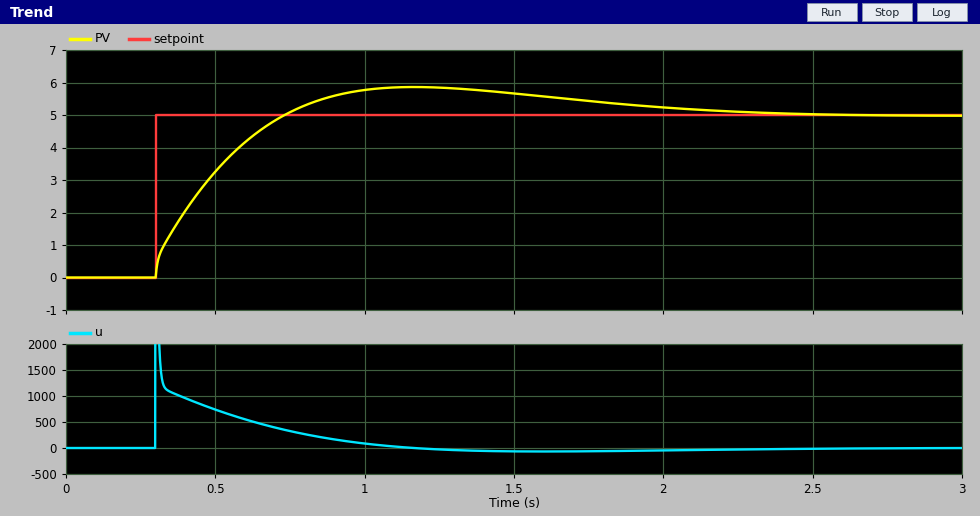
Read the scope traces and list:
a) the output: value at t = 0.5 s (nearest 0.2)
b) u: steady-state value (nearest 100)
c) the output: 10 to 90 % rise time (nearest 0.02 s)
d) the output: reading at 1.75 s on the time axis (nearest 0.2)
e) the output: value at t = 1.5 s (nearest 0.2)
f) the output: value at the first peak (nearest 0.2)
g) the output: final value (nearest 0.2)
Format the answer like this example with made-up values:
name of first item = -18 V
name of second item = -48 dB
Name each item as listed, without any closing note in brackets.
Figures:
the output: value at t = 0.5 s = 3.2
u: steady-state value = 0
the output: 10 to 90 % rise time = 0.34 s
the output: reading at 1.75 s on the time axis = 5.4
the output: value at t = 1.5 s = 5.6
the output: value at the first peak = 5.8
the output: final value = 5.0
